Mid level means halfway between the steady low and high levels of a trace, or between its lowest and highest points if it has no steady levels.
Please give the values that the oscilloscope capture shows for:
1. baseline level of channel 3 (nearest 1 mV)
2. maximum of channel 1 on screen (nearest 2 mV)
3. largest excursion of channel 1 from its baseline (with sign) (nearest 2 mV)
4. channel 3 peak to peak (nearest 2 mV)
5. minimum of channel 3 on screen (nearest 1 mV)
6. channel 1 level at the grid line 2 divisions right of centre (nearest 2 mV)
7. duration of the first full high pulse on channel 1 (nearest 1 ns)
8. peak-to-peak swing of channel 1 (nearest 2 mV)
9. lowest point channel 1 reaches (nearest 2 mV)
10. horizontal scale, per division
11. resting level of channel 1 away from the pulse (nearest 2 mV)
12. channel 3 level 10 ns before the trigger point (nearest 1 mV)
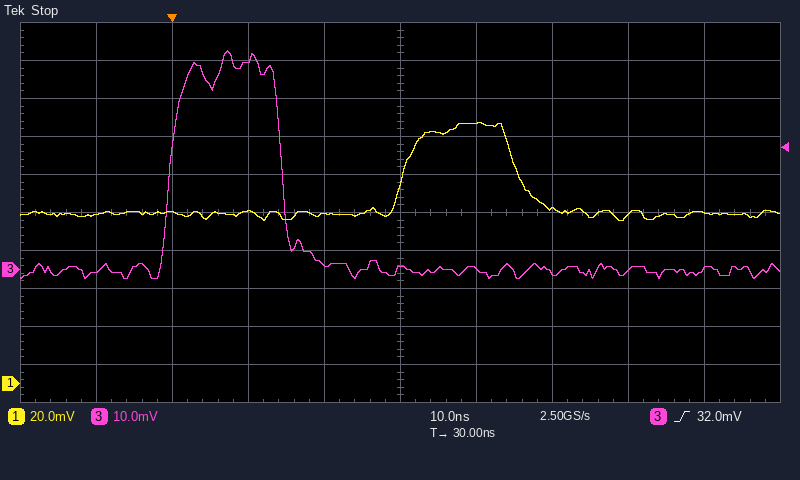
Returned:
0 mV
138 mV
+48 mV
60 mV
-2 mV
92 mV
15 ns
52 mV
86 mV
10 ns
90 mV
0 mV
